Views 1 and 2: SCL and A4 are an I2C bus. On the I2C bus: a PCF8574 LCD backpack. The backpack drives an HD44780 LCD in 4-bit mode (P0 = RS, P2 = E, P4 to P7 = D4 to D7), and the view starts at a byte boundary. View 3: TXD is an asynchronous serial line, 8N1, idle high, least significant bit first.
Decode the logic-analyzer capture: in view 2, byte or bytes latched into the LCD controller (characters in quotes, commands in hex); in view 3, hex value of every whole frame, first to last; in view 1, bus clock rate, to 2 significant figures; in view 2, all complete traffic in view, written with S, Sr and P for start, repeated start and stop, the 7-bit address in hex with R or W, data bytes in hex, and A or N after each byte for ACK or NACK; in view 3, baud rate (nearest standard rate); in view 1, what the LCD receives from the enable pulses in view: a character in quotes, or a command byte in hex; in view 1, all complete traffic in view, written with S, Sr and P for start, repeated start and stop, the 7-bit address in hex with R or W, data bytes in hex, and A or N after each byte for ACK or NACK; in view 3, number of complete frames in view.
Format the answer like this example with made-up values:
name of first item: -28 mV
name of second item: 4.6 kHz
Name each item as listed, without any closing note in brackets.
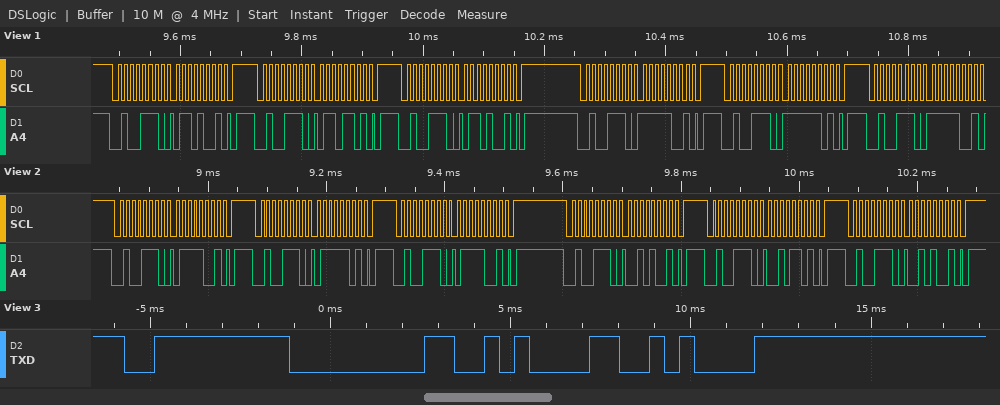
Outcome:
in view 2, byte or bytes latched into the LCD controller: 'r'
in view 3, hex value of every whole frame, first to last: FE 00 0A 0A
in view 1, bus clock rate, to 2 significant figures: 100 kHz
in view 2, all complete traffic in view, written with S, Sr and P for start, repeated start and stop, the 7-bit address in hex with R or W, data bytes in hex, and A or N after each byte for ACK or NACK: S 27W A 79 A P S 27W A 7D A P S 27W A 79 A P S 27W A 29 A P S 27W A 2D A P S 27W A 29 A P
in view 3, baud rate: 2400 baud
in view 1, what the LCD receives from the enable pulses in view: a character in quotes, or a command byte in hex: 'o'
in view 1, all complete traffic in view, written with S, Sr and P for start, repeated start and stop, the 7-bit address in hex with R or W, data bytes in hex, and A or N after each byte for ACK or NACK: S 27W A 69 A P S 27W A 6D A P S 27W A 69 A P S 27W A F9 A P S 27W A FD A P S 27W A F9 A
in view 3, number of complete frames in view: 4
